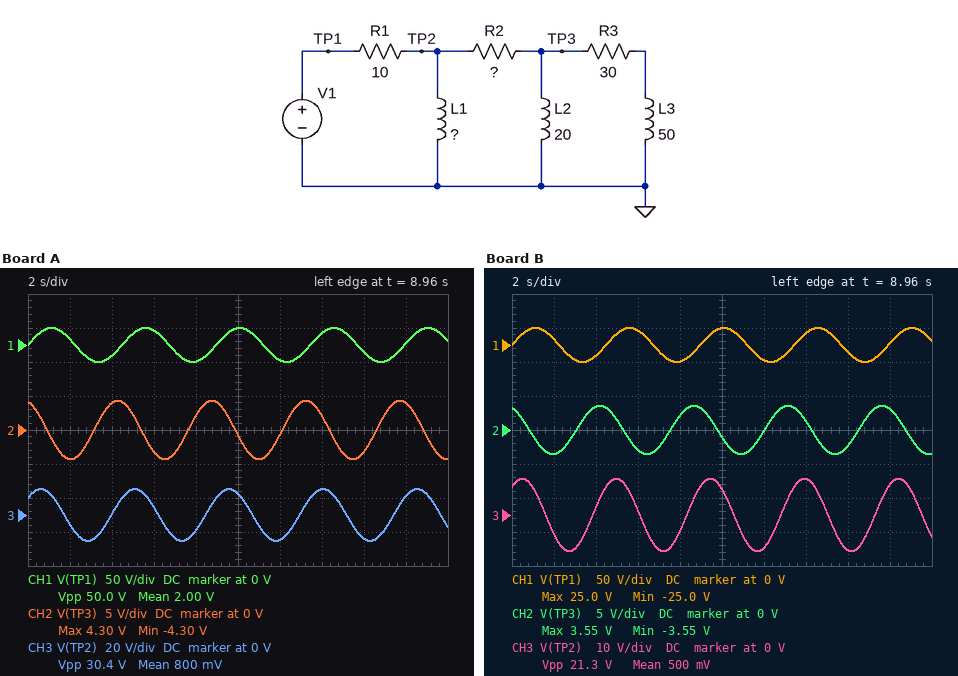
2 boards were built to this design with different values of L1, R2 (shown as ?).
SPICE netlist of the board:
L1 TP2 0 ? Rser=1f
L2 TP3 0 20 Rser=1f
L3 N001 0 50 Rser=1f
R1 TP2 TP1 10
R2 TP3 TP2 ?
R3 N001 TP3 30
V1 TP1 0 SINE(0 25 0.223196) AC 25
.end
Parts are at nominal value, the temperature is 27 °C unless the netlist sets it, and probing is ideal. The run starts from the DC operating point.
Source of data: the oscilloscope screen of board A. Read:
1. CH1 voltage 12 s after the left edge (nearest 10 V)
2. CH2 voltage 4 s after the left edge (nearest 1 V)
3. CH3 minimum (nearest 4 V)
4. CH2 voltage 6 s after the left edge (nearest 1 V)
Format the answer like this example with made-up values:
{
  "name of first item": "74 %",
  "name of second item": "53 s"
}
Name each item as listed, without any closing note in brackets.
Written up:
{
  "CH1 voltage 12 s after the left edge": "-20 V",
  "CH2 voltage 4 s after the left edge": "4 V",
  "CH3 minimum": "-16 V",
  "CH2 voltage 6 s after the left edge": "-3 V"
}
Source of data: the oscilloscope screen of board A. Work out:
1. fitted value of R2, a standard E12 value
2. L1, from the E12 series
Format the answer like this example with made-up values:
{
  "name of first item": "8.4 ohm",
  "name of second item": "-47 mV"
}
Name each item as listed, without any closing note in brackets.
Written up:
{
  "fitted value of R2, a standard E12 value": "68 Ω",
  "L1, from the E12 series": "6.8 H"
}
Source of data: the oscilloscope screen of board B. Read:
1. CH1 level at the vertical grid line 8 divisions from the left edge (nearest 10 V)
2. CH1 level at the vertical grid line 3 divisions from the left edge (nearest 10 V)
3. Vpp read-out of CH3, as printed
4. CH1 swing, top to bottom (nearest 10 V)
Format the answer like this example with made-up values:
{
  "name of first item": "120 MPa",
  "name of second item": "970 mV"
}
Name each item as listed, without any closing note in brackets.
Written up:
{
  "CH1 level at the vertical grid line 8 divisions from the left edge": "-10 V",
  "CH1 level at the vertical grid line 3 divisions from the left edge": "20 V",
  "Vpp read-out of CH3, as printed": "21.3 V",
  "CH1 swing, top to bottom": "50 V"
}
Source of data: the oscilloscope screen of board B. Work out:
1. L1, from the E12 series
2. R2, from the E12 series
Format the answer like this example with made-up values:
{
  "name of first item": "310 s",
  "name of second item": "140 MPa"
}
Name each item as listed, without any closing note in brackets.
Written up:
{
  "L1, from the E12 series": "3.9 H",
  "R2, from the E12 series": "56 Ω"
}
